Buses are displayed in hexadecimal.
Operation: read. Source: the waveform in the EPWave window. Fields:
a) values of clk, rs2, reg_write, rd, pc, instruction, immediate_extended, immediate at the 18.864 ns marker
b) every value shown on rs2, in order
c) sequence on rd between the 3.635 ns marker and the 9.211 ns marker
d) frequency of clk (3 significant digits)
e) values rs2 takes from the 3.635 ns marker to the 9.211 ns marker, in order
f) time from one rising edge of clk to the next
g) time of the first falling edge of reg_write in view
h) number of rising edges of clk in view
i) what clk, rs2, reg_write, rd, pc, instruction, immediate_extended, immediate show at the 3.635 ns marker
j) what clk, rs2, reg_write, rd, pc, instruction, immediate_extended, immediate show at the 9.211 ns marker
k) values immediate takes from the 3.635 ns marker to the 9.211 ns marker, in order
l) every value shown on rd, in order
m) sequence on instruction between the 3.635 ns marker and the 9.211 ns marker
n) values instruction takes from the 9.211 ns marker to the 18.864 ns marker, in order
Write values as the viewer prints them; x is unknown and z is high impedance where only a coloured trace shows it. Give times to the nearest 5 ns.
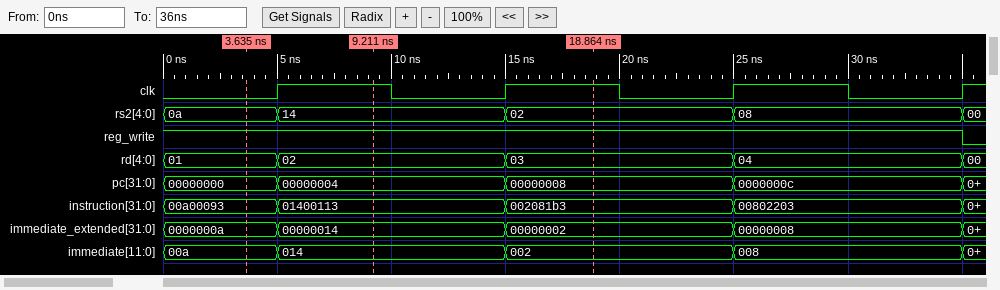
clk=1, rs2=02, reg_write=1, rd=03, pc=00000008, instruction=002081b3, immediate_extended=00000002, immediate=002
0a, 14, 02, 08, 00
01, 02
100 MHz
0a, 14
10 ns
35 ns
4
clk=0, rs2=0a, reg_write=1, rd=01, pc=00000000, instruction=00a00093, immediate_extended=0000000a, immediate=00a
clk=1, rs2=14, reg_write=1, rd=02, pc=00000004, instruction=01400113, immediate_extended=00000014, immediate=014
00a, 014
01, 02, 03, 04, 00
00a00093, 01400113
01400113, 002081b3
